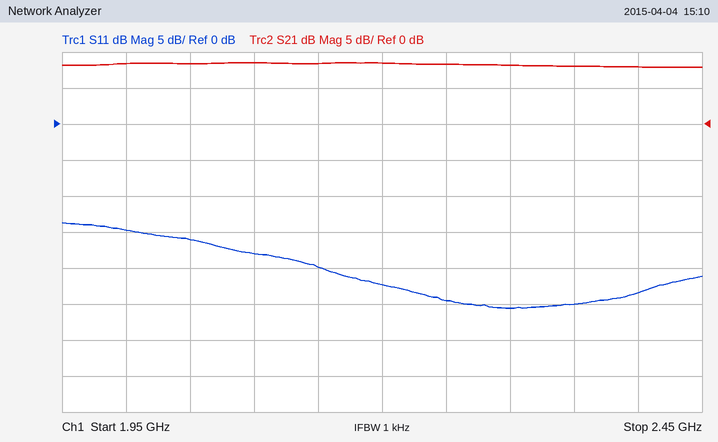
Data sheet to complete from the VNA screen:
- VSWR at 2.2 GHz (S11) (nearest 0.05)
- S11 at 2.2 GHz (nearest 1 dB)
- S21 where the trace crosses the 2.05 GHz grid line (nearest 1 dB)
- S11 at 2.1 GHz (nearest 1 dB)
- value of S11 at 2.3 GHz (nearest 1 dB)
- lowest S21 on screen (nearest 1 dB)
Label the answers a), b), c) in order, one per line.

a) 1.15
b) -22 dB
c) 8 dB
d) -18 dB
e) -26 dB
f) 8 dB
